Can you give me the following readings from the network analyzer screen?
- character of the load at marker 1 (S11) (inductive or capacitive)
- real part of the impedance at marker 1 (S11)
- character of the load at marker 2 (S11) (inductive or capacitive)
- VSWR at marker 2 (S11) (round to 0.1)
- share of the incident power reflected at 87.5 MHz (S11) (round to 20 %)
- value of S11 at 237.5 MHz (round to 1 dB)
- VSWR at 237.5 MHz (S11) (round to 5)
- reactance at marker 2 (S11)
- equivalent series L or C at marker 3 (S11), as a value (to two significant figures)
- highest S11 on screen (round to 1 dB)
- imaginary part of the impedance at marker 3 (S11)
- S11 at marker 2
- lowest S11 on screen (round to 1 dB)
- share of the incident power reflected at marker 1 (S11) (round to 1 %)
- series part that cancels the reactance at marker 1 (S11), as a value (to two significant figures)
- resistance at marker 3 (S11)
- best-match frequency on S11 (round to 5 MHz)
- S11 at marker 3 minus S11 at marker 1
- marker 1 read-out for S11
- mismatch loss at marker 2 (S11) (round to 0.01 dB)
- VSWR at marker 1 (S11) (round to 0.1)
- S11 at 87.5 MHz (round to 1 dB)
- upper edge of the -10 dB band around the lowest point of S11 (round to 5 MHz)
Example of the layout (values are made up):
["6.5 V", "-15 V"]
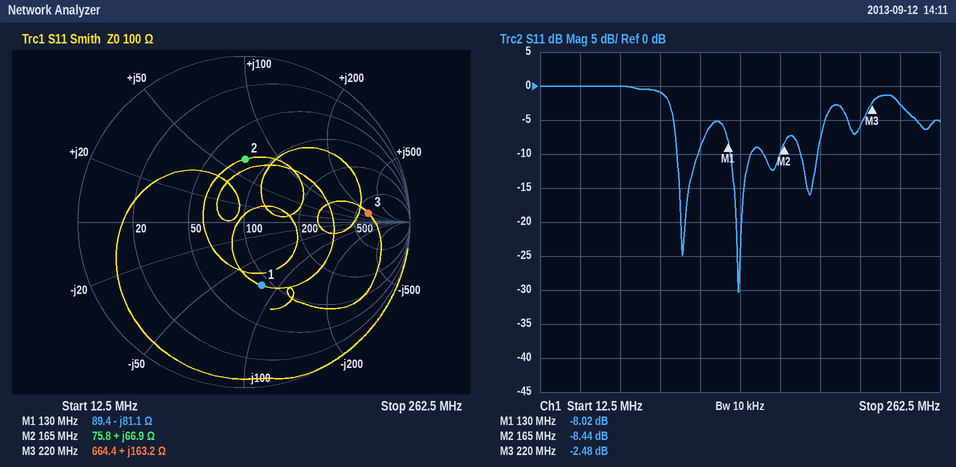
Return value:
["capacitive", "89.4 Ω", "inductive", "2.2", "80 %", "-3 dB", "5", "+66.9 Ω", "120 nH", "0 dB", "+163.2 Ω", "-8.44 dB", "-30 dB", "16 %", "99 nH", "664.4 Ω", "135 MHz", "5.54 dB", "-8.02 dB", "0.67 dB", "2.3", "-1 dB", "145 MHz"]
